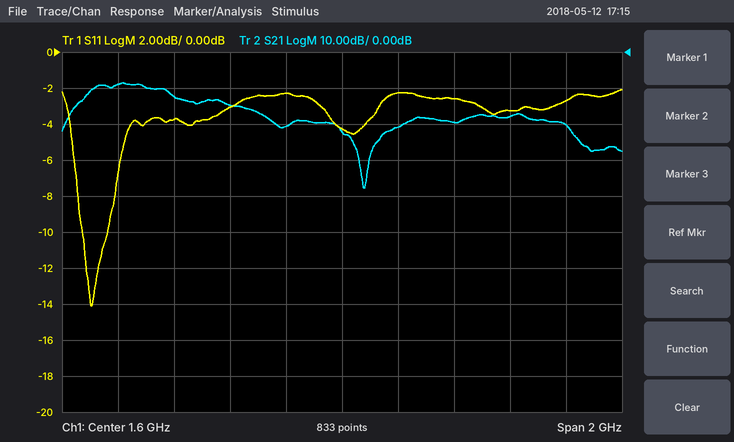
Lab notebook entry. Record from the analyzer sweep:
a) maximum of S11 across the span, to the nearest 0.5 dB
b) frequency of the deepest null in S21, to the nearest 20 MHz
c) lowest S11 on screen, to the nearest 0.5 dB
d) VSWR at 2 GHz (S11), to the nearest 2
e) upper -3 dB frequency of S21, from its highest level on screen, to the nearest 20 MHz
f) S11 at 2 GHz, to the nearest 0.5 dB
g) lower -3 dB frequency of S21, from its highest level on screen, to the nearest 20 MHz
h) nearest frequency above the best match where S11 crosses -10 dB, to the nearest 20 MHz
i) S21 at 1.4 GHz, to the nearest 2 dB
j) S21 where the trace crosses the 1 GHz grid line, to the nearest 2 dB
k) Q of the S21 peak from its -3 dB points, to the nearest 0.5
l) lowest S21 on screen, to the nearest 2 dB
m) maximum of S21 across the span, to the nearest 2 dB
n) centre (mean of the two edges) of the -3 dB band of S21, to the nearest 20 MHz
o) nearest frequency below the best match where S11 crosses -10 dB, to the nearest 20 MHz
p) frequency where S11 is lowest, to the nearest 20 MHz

-2.0 dB
1.68 GHz
-14.0 dB
6
980 MHz
-2.5 dB
700 MHz
760 MHz
-20 dB
-12 dB
3.0
-38 dB
-8 dB
840 MHz
680 MHz
700 MHz
